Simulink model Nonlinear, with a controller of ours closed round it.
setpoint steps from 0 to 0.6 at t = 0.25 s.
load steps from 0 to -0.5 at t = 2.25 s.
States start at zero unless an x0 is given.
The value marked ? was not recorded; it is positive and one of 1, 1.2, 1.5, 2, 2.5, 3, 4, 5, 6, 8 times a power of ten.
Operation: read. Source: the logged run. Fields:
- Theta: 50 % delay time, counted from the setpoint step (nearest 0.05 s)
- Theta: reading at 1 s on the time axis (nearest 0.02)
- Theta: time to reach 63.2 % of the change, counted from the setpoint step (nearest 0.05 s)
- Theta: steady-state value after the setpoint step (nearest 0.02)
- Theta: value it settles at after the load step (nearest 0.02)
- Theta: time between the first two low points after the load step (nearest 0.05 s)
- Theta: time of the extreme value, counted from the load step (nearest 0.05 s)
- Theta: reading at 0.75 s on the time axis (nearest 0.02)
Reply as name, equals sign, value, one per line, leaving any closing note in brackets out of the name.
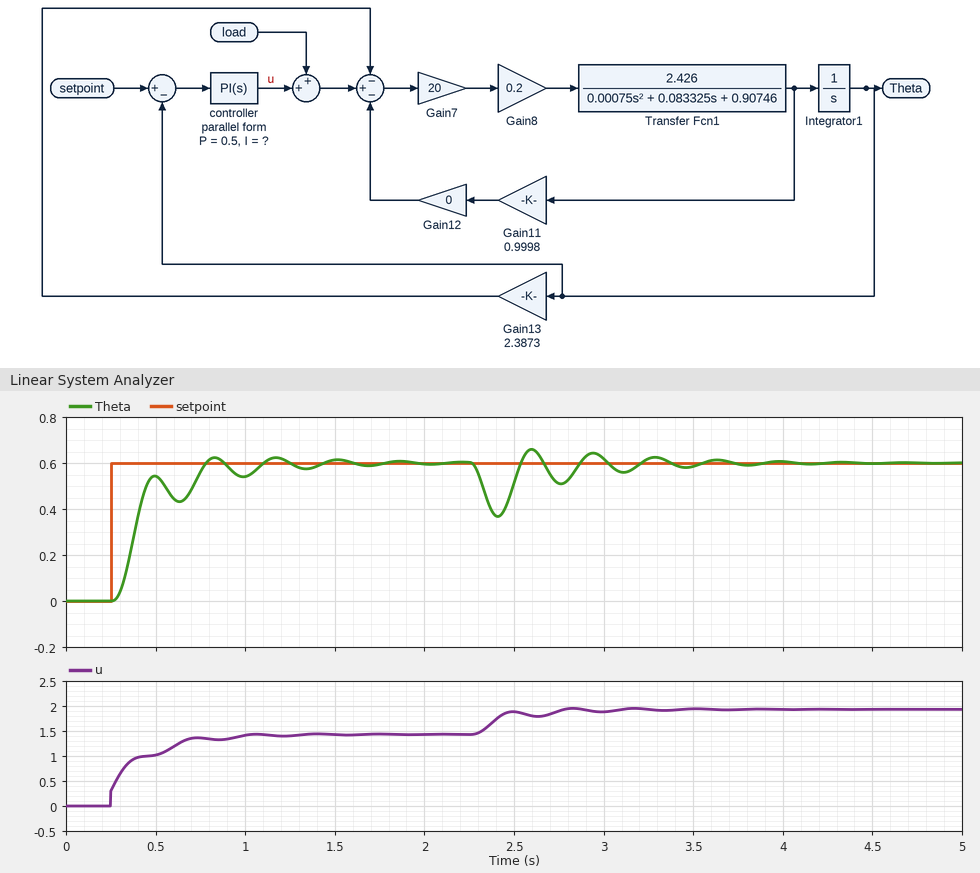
Theta: 50 % delay time, counted from the setpoint step = 0.15 s
Theta: reading at 1 s on the time axis = 0.54
Theta: time to reach 63.2 % of the change, counted from the setpoint step = 0.15 s
Theta: steady-state value after the setpoint step = 0.60
Theta: value it settles at after the load step = 0.60
Theta: time between the first two low points after the load step = 0.35 s
Theta: time of the extreme value, counted from the load step = 0.15 s
Theta: reading at 0.75 s on the time axis = 0.56
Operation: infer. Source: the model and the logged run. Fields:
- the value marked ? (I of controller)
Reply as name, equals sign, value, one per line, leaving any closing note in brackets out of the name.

the value marked ? = 12
